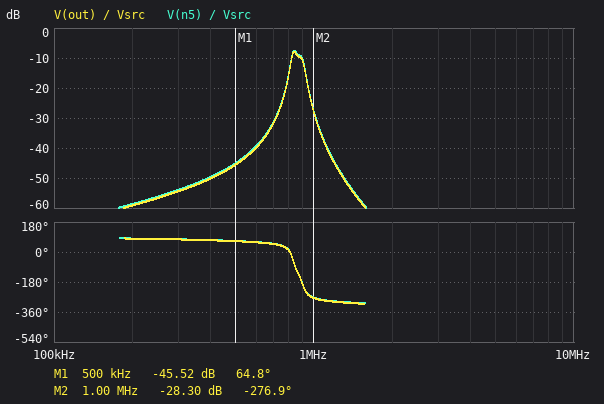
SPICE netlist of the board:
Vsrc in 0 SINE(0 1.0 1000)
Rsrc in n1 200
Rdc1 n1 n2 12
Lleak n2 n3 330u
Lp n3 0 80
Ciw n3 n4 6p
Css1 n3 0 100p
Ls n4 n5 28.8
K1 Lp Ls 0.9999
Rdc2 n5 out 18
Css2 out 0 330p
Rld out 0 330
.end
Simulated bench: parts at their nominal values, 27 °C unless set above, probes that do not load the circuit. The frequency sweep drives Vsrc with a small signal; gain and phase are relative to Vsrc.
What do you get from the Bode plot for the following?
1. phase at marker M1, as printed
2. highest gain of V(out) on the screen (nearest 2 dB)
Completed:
64.8 deg
-8 dB
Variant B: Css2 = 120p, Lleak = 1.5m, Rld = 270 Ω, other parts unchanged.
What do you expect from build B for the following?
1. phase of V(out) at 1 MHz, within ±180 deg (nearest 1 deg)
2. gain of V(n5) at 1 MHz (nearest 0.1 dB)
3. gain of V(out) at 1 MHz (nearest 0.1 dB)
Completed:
82 deg
-52.2 dB
-52.7 dB
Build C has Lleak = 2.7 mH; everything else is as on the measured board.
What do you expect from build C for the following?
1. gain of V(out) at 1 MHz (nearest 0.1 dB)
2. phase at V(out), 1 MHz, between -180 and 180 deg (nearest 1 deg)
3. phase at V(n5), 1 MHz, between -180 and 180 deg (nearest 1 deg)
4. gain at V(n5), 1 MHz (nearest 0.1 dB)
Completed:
-58.3 dB
58 deg
60 deg
-57.8 dB
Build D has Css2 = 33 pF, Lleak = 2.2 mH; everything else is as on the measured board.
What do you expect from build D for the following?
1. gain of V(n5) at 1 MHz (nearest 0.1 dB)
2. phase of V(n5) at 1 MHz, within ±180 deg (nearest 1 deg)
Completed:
-54.3 dB
89 deg
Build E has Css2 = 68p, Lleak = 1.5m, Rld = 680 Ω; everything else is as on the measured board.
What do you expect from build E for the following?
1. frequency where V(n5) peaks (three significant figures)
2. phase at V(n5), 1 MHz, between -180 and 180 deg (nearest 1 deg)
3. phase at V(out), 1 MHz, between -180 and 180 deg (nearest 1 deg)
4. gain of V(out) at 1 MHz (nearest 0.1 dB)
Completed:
863 kHz
80 deg
79 deg
-44.8 dB
